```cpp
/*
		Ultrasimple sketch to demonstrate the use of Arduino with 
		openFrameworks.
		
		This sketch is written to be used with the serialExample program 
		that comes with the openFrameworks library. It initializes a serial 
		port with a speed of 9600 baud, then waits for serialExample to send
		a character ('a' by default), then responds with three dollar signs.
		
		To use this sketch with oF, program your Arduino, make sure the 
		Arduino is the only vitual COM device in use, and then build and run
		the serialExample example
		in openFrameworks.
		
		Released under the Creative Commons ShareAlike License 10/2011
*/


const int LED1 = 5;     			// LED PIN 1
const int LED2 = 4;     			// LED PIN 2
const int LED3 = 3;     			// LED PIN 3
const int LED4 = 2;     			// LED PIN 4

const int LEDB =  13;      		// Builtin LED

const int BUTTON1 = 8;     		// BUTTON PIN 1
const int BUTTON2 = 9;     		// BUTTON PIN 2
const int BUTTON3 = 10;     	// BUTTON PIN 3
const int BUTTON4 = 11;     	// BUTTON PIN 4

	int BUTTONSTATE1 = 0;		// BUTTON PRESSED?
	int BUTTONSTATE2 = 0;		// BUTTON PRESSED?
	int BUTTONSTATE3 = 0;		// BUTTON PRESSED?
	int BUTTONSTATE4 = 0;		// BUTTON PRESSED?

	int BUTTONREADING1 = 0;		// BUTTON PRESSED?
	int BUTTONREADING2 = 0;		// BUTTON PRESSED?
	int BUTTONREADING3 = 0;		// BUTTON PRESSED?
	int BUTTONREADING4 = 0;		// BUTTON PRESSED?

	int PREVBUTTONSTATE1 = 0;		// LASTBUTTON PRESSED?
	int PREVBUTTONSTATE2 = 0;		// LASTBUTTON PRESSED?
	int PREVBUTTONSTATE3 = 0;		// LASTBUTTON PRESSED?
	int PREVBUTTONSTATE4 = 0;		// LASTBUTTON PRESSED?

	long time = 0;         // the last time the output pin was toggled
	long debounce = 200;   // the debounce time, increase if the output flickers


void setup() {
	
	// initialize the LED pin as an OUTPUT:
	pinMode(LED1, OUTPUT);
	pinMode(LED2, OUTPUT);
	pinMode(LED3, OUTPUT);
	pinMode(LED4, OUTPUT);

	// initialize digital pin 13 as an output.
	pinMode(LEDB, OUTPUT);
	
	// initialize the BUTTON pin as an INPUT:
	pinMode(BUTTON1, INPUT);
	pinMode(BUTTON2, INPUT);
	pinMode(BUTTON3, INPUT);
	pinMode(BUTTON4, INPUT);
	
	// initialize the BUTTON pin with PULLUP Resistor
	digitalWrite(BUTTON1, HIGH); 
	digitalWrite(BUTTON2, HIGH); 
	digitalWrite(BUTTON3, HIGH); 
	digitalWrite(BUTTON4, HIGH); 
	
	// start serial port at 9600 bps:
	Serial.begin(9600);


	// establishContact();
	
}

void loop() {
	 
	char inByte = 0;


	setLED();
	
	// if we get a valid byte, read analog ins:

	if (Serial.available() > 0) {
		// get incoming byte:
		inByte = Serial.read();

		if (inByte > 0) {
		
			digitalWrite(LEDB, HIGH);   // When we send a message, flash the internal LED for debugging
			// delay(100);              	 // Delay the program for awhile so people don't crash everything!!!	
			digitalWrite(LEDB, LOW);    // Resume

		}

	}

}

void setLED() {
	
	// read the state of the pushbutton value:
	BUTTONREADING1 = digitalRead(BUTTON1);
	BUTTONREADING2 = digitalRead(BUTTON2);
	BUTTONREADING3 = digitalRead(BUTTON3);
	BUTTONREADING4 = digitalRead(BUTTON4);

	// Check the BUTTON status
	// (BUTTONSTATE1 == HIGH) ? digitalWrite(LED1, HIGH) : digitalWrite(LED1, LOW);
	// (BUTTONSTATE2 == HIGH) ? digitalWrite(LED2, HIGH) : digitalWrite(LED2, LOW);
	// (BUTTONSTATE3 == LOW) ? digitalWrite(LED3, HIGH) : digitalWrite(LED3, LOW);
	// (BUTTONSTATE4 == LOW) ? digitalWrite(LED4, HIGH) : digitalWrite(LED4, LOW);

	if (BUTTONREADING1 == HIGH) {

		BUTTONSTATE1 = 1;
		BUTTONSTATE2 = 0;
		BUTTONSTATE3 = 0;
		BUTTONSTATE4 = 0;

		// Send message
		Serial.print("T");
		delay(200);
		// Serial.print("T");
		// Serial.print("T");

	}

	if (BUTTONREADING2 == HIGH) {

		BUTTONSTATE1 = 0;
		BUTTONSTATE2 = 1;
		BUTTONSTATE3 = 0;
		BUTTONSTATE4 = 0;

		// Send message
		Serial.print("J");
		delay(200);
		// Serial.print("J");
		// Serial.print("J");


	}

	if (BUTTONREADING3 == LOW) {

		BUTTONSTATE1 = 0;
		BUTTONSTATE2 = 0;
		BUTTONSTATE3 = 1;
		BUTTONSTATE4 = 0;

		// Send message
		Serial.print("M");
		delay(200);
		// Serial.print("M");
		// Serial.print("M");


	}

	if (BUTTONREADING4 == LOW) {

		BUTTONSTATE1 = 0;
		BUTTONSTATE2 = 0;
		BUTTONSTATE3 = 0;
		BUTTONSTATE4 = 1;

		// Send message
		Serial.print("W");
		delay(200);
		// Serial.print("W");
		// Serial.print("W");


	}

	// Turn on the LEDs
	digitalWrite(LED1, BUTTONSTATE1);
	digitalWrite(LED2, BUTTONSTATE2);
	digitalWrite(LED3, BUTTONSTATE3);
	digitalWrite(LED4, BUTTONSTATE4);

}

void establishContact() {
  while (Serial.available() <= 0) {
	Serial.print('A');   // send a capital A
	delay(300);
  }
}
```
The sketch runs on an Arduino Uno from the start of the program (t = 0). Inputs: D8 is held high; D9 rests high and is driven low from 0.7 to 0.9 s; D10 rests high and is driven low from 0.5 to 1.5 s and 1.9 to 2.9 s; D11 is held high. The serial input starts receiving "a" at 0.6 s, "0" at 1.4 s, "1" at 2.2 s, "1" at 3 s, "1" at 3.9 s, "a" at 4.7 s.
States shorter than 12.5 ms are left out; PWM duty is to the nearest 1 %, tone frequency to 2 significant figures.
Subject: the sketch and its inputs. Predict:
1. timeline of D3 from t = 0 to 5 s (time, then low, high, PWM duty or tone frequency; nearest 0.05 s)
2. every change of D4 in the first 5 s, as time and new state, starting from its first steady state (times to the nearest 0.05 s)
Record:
0 s low; 1.2 s high; 2.2 s low; 2.8 s high; 3.8 s low
0 s low; 0.4 s high; 1.2 s low; 2.2 s high; 2.8 s low; 3.8 s high
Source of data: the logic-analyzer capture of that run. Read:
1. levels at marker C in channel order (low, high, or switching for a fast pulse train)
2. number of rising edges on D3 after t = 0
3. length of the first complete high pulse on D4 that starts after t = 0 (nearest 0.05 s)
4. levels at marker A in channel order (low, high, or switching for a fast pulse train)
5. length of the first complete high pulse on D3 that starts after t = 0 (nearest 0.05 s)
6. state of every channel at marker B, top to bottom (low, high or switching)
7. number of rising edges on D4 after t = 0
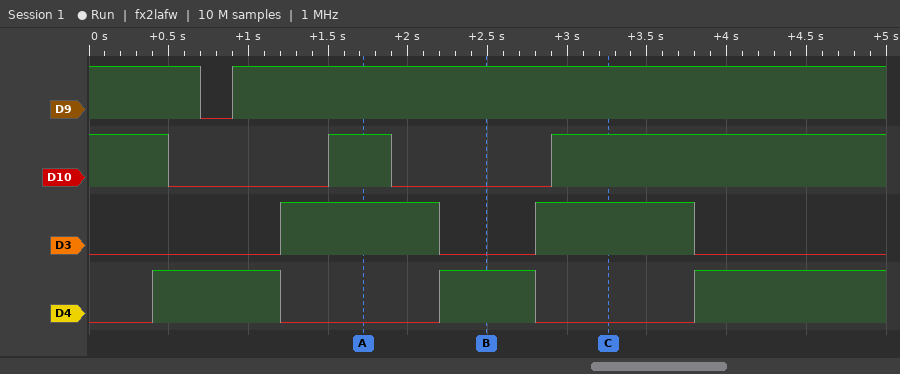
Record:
D9 high, D10 high, D3 high, D4 low
2
0.80 s
D9 high, D10 high, D3 high, D4 low
1.00 s
D9 high, D10 low, D3 low, D4 high
3
